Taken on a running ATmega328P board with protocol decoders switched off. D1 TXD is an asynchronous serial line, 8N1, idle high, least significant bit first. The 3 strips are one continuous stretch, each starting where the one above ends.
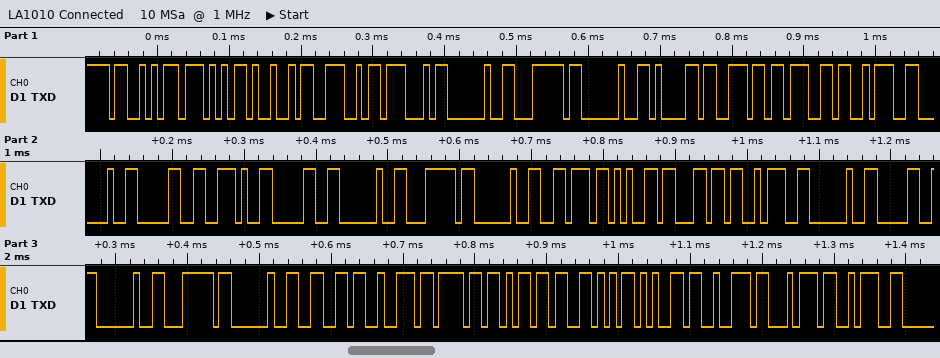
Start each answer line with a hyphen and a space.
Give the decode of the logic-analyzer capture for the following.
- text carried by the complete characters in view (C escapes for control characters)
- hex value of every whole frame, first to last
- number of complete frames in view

- "SWING | ang: 0.0 | vel: 0 | fromVert:"
- 53 57 49 4E 47 20 7C 20 61 6E 67 3A 20 30 2E 30 20 7C 20 76 65 6C 3A 20 30 20 7C 20 66 72 6F 6D 56 65 72 74 3A
- 37
